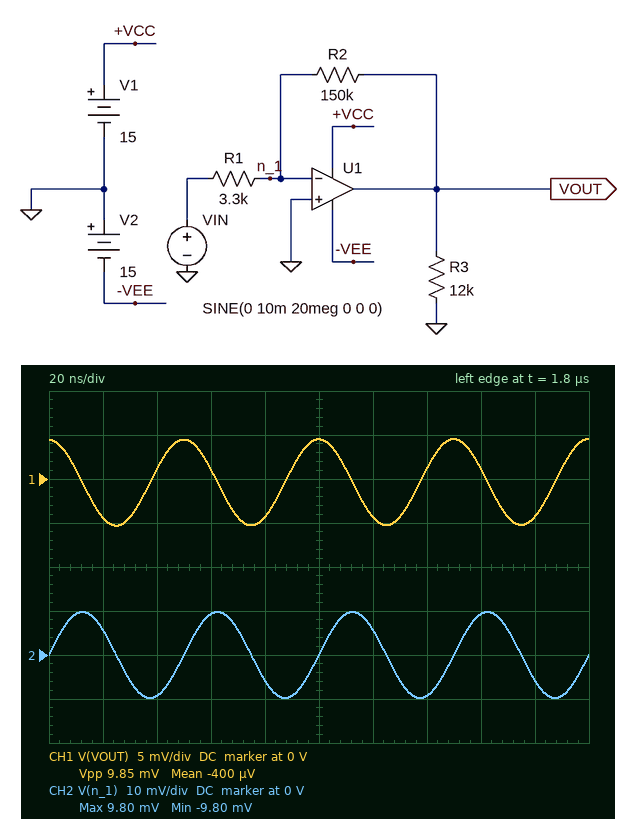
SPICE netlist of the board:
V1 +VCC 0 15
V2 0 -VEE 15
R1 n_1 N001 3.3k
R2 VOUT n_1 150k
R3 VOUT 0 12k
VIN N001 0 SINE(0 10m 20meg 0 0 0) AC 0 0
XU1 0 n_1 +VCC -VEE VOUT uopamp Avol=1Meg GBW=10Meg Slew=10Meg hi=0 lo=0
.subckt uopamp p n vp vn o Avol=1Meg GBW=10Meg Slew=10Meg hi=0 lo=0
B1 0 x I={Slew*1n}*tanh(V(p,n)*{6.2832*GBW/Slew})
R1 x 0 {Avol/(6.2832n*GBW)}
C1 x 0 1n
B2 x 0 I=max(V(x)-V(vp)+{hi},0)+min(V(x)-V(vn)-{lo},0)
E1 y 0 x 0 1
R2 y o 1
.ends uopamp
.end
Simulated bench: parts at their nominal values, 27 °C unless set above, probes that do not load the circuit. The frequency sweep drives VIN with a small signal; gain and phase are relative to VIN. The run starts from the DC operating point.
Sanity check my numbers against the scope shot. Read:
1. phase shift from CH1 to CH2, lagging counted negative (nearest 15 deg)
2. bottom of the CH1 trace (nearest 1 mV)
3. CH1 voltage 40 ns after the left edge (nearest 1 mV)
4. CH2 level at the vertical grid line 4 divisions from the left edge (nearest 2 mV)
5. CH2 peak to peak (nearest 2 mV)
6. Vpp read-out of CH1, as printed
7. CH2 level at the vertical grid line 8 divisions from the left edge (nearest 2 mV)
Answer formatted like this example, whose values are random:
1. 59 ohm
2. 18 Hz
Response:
1. -90 deg
2. -5 mV
3. 1 mV
4. -6 mV
5. 20 mV
6. 9.85 mV
7. 10 mV
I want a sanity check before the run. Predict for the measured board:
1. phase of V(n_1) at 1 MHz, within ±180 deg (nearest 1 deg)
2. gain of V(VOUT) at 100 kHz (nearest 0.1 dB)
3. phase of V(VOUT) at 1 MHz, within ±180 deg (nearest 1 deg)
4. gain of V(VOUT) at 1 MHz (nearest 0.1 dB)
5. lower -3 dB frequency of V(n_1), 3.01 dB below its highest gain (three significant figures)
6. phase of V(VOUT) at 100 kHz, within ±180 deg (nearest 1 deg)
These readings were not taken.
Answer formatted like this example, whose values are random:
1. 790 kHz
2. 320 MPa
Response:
1. 12 deg
2. 32.3 dB
3. 102 deg
4. 19.6 dB
5. 215 kHz
6. 155 deg
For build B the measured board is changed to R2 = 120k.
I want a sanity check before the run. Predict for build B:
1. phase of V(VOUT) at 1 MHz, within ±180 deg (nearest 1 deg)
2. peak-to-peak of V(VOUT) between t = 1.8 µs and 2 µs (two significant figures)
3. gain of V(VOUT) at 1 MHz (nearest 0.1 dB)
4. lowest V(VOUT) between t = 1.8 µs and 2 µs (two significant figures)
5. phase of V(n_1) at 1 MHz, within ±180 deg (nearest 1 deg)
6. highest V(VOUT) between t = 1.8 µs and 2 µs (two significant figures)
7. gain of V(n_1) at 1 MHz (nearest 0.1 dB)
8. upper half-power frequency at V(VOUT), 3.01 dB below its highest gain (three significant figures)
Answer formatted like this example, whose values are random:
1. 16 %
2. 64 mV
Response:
1. 105 deg
2. 9.8 mV
3. 19.5 dB
4. -5.1 mV
5. 15 deg
6. 4.7 mV
7. -0.5 dB
8. 268 kHz
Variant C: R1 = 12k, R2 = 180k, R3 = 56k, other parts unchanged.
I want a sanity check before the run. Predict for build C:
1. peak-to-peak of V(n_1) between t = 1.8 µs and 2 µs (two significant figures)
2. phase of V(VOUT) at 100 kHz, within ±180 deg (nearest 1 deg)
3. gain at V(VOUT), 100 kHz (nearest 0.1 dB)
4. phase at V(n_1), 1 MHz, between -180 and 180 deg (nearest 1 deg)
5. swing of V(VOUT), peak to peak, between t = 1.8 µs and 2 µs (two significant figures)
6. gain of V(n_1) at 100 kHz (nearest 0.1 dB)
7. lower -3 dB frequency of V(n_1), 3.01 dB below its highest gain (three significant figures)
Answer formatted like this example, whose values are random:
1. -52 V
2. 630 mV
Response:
1. 19 mV
2. 171 deg
3. 23.4 dB
4. 32 deg
5. 9.4 mV
6. -16.6 dB
7. 625 kHz
